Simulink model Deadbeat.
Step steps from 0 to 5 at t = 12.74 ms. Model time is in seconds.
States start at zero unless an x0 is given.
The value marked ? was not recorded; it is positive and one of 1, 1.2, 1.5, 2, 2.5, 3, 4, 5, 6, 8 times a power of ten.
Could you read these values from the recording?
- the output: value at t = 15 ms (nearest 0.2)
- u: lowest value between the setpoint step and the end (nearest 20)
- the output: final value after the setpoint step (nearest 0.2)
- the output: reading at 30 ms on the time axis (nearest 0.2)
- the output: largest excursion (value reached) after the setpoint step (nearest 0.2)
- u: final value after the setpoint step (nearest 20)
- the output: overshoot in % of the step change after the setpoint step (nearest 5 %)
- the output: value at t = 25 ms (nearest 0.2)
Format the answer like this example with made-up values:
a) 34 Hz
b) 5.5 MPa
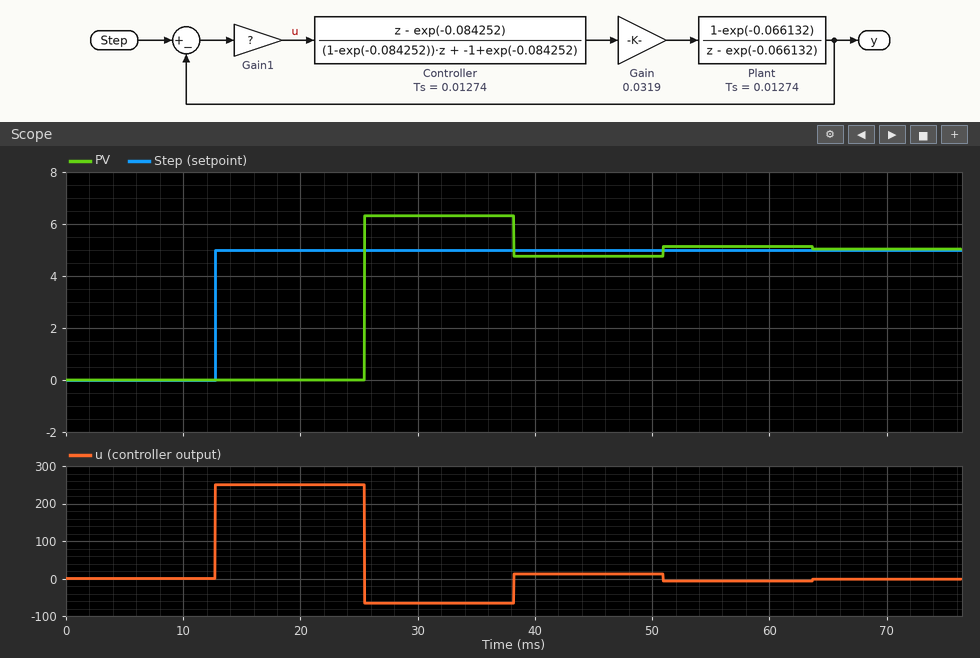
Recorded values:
a) 0.0
b) -60
c) 5.0
d) 6.4
e) 6.4
f) 0
g) 25 %
h) 0.0
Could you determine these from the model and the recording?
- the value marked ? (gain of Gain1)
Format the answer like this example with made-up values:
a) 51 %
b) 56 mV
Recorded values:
a) 50
